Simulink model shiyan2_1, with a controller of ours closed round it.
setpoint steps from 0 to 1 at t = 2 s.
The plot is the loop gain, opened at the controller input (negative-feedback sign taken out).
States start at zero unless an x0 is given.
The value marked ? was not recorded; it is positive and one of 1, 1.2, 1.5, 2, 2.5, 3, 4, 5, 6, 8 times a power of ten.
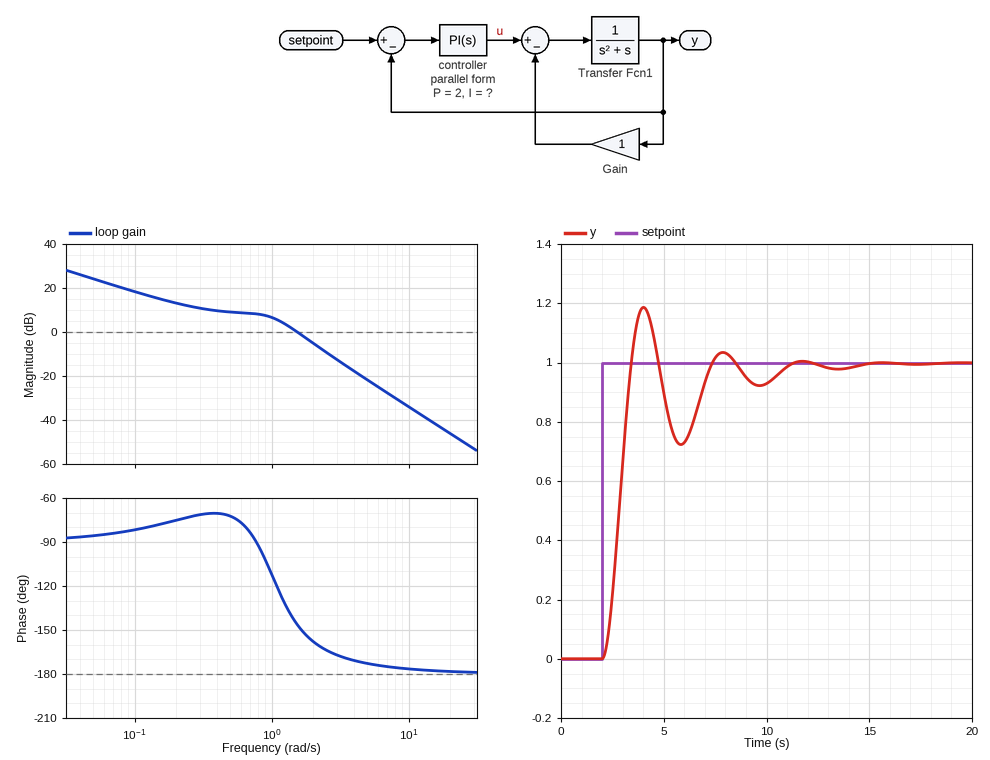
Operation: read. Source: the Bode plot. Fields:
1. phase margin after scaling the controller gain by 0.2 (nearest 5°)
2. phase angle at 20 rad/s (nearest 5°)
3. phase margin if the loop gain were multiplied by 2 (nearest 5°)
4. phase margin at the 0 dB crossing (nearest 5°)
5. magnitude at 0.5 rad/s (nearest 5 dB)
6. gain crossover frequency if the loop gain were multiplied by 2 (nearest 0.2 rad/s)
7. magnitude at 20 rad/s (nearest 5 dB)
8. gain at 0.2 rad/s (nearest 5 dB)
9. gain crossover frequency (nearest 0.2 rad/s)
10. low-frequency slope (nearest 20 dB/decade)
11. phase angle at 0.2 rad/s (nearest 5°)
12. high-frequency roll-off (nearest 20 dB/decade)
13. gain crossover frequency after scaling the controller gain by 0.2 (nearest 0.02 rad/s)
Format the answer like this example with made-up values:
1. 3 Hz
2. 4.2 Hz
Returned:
1. 105°
2. -180°
3. 20°
4. 35°
5. 10 dB
6. 2.2 rad/s
7. -45 dB
8. 15 dB
9. 1.6 rad/s
10. -20 dB/decade
11. -75°
12. -40 dB/decade
13. 0.18 rad/s
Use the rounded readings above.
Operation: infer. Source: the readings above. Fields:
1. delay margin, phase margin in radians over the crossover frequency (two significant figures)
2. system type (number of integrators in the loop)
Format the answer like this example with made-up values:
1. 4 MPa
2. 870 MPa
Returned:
1. 0.38 s
2. 1
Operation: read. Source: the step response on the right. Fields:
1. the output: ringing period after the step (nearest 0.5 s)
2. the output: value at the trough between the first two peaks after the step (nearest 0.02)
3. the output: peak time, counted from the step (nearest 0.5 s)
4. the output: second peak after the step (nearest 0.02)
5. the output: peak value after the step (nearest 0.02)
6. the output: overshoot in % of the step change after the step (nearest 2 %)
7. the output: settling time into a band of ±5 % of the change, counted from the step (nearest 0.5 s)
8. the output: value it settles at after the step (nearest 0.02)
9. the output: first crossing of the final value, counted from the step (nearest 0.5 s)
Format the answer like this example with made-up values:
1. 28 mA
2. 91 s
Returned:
1. 4.0 s
2. 0.72
3. 2.0 s
4. 1.04
5. 1.18
6. 18 %
7. 8.5 s
8. 1.00
9. 1.5 s
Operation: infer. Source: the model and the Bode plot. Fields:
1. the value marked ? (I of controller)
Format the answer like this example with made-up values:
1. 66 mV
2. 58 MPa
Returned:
1. 0.8
